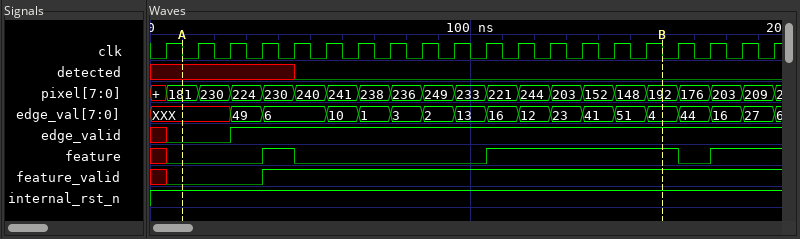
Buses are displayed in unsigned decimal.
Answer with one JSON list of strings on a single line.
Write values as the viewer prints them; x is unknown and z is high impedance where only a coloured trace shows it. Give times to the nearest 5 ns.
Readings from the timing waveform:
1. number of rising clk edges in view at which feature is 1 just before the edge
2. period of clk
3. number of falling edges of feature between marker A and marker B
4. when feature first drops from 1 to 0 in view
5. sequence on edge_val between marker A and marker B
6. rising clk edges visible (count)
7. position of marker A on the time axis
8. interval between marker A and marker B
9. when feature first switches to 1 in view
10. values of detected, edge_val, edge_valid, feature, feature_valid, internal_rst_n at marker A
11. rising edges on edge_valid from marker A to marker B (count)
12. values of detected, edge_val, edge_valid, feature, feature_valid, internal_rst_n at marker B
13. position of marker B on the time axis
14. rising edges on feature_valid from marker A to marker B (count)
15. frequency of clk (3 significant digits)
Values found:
["9", "10 ns", "1", "45 ns", "XXX, 49, 6, 10, 1, 3, 2, 13, 16, 12, 23, 41, 51, 4", "20", "10 ns", "150 ns", "35 ns", "detected=x, edge_val=XXX, edge_valid=0, feature=0, feature_valid=0, internal_rst_n=1", "1", "detected=0, edge_val=4, edge_valid=1, feature=1, feature_valid=1, internal_rst_n=1", "160 ns", "1", "100 MHz"]
